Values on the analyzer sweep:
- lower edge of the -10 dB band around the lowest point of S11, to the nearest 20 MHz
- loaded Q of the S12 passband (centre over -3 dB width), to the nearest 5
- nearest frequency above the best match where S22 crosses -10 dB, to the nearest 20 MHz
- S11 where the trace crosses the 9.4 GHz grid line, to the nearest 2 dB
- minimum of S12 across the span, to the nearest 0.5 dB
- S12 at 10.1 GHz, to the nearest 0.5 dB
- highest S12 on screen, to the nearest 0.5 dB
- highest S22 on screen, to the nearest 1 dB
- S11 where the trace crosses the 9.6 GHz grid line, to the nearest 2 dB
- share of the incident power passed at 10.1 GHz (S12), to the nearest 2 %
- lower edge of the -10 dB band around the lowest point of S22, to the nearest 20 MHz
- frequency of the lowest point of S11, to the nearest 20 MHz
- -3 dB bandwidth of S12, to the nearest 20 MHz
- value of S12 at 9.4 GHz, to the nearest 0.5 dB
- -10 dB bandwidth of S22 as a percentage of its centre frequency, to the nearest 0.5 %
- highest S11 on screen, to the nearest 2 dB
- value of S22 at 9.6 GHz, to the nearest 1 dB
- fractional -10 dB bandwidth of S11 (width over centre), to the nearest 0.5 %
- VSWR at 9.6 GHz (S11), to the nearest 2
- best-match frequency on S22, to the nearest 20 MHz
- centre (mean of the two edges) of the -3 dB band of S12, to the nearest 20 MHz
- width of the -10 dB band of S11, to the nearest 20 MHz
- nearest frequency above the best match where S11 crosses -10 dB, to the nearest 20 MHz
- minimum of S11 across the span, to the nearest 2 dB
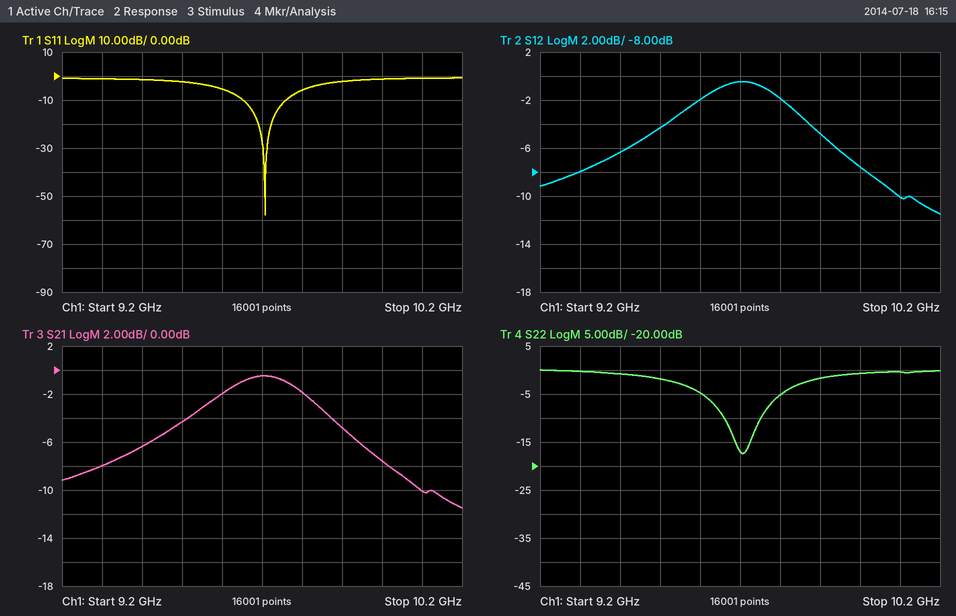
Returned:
9.66 GHz
30
9.76 GHz
-2 dB
-11.5 dB
-10.0 dB
-0.5 dB
0 dB
-6 dB
10 %
9.66 GHz
9.70 GHz
320 MHz
-6.5 dB
1.0 %
0 dB
-5 dB
1.0 %
4
9.70 GHz
9.70 GHz
100 MHz
9.76 GHz
-58 dB
